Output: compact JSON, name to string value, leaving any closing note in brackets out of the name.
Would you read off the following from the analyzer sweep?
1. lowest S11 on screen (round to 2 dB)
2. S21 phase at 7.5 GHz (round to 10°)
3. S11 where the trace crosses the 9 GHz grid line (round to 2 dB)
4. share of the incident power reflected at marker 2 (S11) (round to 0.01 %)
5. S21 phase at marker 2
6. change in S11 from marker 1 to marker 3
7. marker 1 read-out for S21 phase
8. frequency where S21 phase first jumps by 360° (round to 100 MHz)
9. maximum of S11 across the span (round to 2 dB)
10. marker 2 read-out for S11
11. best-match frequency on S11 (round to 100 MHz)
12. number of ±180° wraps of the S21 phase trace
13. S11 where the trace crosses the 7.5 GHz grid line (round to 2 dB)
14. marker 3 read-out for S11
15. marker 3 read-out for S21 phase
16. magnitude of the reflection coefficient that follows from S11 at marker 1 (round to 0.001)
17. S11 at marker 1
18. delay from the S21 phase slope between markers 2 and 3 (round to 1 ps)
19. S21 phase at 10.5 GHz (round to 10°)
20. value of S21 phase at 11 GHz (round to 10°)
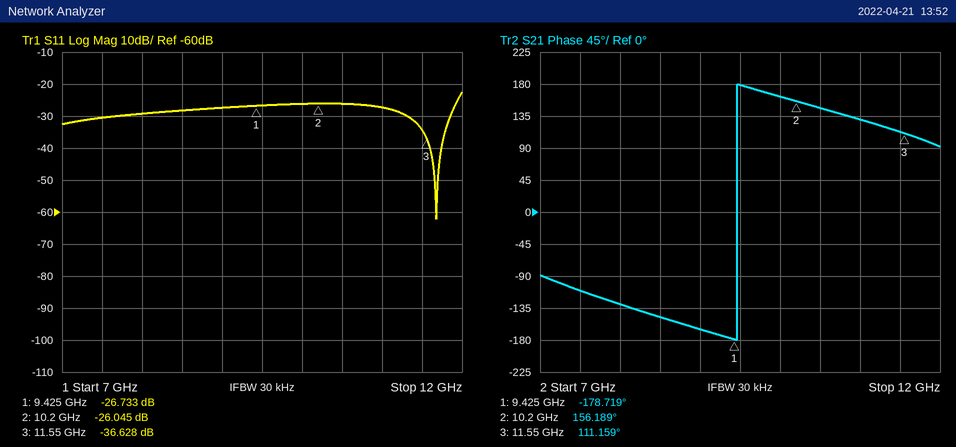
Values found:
{"lowest S11 on screen": "-62 dB", "S21 phase at 7.5 GHz": "-110°", "S11 where the trace crosses the 9 GHz grid line": "-28 dB", "share of the incident power reflected at marker 2 (S11)": "0.25 %", "S21 phase at marker 2": "156.189°", "change in S11 from marker 1 to marker 3": "-9.895 dB", "marker 1 read-out for S21 phase": "-178.719°", "frequency where S21 phase first jumps by 360°": "9.5 GHz", "maximum of S11 across the span": "-22 dB", "marker 2 read-out for S11": "-26.045 dB", "best-match frequency on S11": "11.7 GHz", "number of ±180° wraps of the S21 phase trace": "1", "S11 where the trace crosses the 7.5 GHz grid line": "-30 dB", "marker 3 read-out for S11": "-36.628 dB", "marker 3 read-out for S21 phase": "111.159°", "magnitude of the reflection coefficient that follows from S11 at marker 1": "0.046", "S11 at marker 1": "-26.733 dB", "delay from the S21 phase slope between markers 2 and 3": "93 ps", "S21 phase at 10.5 GHz": "150°", "value of S21 phase at 11 GHz": "130°"}
